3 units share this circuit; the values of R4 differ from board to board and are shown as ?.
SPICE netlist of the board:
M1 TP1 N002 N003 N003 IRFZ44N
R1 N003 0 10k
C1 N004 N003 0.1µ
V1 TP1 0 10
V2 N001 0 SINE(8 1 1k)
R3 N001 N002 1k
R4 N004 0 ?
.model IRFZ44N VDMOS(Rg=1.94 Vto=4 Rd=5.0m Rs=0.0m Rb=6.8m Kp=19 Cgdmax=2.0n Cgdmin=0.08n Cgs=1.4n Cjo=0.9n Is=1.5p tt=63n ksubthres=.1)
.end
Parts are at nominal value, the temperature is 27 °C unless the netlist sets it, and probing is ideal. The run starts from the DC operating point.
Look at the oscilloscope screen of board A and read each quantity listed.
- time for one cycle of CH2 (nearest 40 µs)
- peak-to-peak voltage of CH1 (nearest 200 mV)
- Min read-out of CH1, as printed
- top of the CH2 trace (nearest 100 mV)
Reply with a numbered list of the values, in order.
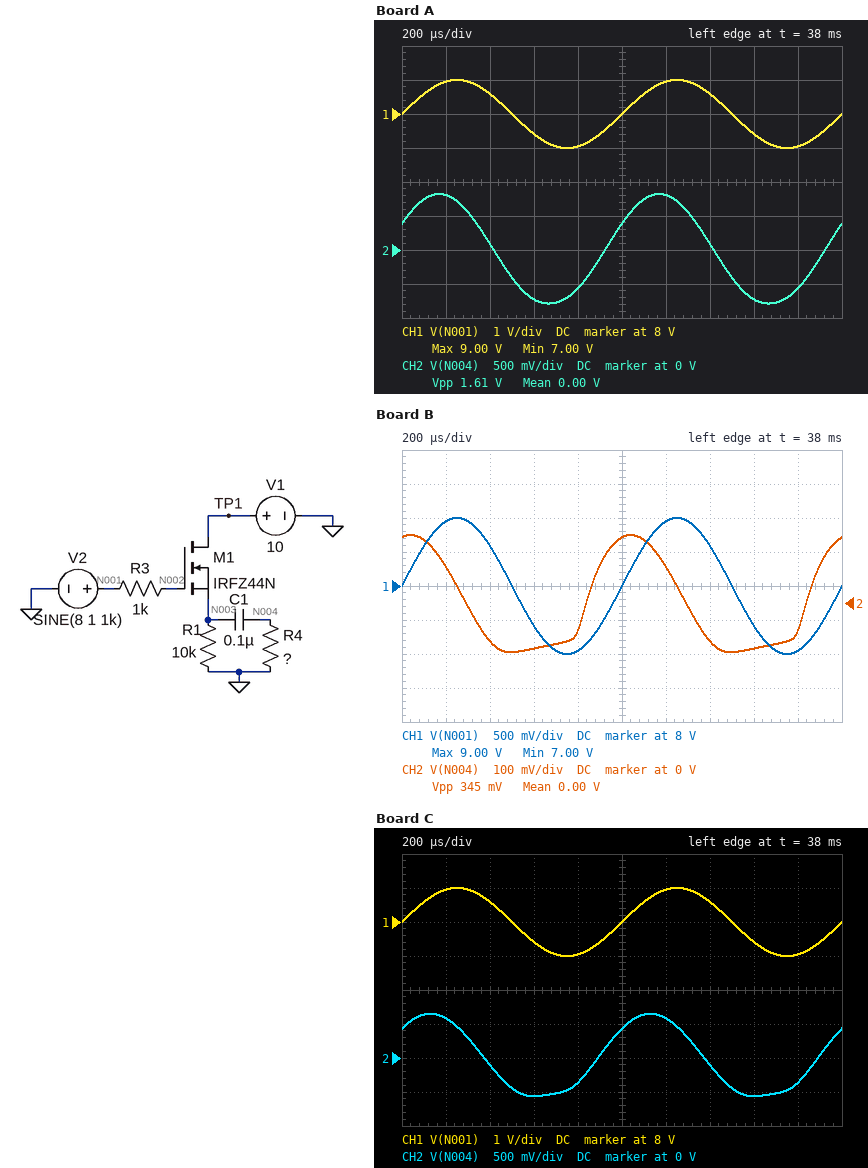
1. 1.00 ms
2. 2.0 V
3. 7.00 V
4. 800 mV
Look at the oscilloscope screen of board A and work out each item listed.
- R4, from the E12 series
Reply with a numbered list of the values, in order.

1. 2.7 kΩ
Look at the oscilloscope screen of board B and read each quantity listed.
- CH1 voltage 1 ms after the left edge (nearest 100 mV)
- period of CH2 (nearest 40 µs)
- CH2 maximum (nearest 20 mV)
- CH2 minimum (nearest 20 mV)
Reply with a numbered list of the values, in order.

1. 8.0 V
2. 1.00 ms
3. 200 mV
4. -140 mV
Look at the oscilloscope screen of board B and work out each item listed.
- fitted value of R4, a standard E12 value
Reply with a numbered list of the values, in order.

1. 330 Ω
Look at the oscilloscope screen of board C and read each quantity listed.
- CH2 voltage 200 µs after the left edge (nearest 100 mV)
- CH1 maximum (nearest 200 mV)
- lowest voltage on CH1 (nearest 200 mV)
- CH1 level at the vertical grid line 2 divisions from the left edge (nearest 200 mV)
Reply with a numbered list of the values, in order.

1. 600 mV
2. 9.0 V
3. 7.0 V
4. 8.6 V
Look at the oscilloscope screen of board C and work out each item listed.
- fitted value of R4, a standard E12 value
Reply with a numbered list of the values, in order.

1. 1.5 kΩ
